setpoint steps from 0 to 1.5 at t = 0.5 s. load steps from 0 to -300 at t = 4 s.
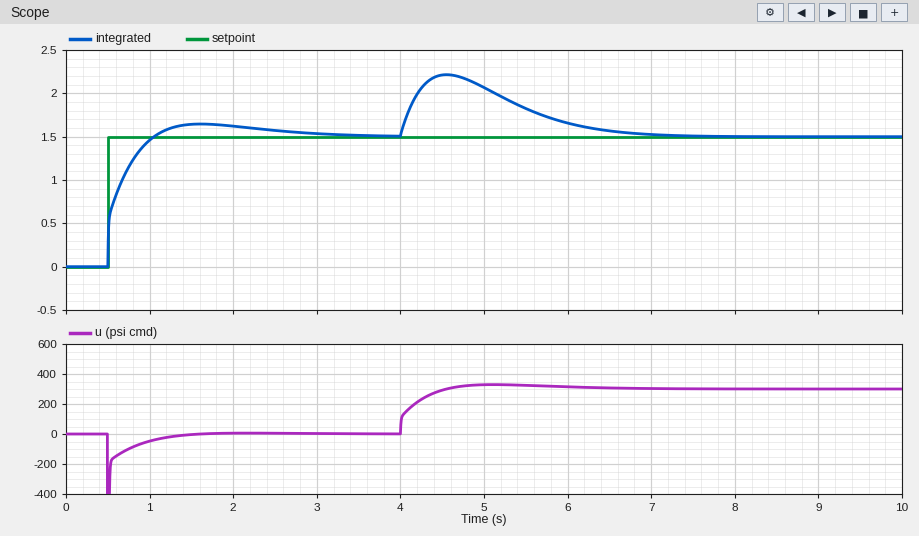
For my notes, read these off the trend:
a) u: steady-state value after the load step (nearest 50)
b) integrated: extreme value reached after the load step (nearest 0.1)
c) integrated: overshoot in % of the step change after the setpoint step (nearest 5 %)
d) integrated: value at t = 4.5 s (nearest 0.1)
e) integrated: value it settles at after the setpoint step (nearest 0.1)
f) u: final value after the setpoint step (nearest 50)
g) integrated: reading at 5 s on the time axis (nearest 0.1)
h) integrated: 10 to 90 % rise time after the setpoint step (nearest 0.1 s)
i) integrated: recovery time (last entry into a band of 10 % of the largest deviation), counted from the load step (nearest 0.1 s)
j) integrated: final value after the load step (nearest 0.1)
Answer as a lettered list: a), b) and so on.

a) 300
b) 2.2
c) 10 %
d) 2.2
e) 1.5
f) 0
g) 2.1
h) 0.4 s
i) 2.5 s
j) 1.5
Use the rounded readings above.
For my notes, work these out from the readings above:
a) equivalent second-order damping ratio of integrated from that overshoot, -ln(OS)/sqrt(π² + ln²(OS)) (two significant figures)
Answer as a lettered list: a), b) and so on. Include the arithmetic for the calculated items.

a) ln(0.1) = -2.303; 2.303 / sqrt(9.870 + 5.302) = 0.59
